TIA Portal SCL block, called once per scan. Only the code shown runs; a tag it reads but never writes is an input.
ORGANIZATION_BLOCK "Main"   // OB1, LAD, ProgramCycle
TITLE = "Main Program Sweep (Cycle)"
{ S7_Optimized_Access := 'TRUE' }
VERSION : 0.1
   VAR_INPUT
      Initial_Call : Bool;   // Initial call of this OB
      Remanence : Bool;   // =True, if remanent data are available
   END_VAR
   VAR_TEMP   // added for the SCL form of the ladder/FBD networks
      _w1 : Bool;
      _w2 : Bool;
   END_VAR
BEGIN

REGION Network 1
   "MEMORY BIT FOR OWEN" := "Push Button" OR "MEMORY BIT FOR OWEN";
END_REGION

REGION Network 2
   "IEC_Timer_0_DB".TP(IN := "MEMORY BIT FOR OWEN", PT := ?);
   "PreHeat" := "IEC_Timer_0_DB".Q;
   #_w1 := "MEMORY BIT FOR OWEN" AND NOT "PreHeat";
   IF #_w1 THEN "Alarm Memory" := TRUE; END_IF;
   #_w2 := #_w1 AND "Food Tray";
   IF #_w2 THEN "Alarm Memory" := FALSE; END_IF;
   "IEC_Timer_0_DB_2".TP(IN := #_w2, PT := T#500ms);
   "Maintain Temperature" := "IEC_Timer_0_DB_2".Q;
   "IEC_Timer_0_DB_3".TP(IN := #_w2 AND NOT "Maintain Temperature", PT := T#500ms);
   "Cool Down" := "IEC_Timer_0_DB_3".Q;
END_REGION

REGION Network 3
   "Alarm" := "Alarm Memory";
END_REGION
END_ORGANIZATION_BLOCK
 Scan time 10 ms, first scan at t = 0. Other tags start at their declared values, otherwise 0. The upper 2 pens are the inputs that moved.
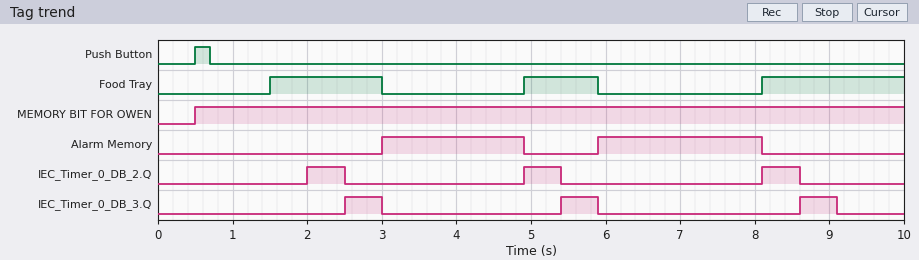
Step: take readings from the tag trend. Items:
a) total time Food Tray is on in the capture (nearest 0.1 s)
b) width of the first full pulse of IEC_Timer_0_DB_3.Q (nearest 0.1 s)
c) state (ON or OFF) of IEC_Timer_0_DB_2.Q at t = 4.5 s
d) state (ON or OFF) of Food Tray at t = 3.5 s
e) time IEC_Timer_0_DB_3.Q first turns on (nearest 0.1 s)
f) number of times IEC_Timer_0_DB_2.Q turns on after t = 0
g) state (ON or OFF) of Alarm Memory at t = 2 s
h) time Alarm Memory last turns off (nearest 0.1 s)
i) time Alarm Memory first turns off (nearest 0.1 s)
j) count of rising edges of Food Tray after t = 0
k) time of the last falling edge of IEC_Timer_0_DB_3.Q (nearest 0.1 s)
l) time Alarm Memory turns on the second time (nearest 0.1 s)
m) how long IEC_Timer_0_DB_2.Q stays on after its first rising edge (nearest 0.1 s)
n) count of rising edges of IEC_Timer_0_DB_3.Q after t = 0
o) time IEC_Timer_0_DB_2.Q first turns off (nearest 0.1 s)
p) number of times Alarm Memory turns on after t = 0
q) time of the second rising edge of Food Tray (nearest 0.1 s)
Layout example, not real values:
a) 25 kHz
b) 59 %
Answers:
a) 4.4 s
b) 0.5 s
c) OFF
d) OFF
e) 2.5 s
f) 3
g) OFF
h) 8.1 s
i) 4.9 s
j) 3
k) 9.1 s
l) 5.9 s
m) 0.5 s
n) 3
o) 2.5 s
p) 2
q) 4.9 s
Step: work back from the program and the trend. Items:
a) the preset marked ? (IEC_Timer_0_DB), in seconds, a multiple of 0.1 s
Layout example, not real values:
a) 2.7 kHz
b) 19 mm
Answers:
a) 1.5 s
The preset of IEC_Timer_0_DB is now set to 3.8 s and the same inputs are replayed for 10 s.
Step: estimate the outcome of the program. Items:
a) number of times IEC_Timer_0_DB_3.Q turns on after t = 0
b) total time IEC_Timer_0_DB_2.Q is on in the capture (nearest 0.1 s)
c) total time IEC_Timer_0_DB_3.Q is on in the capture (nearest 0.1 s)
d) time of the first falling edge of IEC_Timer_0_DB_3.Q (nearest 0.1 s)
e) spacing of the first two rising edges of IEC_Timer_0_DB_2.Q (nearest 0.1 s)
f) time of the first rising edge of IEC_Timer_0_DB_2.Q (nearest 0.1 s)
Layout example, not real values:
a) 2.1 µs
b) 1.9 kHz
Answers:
a) 2
b) 1.0 s
c) 1.0 s
d) 5.9 s
e) 3.2 s
f) 4.9 s
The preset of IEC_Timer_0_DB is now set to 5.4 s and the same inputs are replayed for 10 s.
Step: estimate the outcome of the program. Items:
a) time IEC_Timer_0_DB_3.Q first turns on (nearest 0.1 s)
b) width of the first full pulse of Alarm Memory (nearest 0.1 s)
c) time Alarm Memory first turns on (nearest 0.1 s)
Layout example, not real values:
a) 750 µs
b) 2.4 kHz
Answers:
a) 8.6 s
b) 2.2 s
c) 5.9 s
